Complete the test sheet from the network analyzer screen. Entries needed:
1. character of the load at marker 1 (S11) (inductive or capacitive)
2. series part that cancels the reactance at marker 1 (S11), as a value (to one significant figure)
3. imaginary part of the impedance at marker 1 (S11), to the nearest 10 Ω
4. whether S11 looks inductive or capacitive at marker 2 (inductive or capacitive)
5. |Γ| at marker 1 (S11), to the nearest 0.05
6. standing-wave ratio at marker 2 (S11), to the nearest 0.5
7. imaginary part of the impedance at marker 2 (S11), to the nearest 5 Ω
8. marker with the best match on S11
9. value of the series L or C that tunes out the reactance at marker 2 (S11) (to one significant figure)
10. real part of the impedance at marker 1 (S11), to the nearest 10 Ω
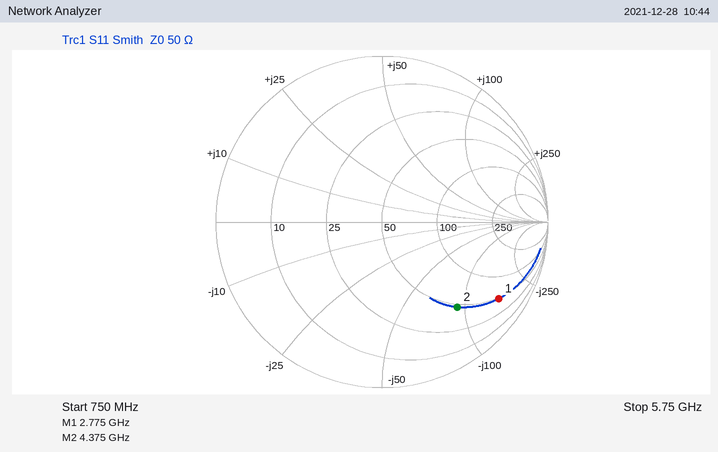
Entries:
capacitive
9 nH
-150 Ω
capacitive
0.85
5.5
-90 Ω
marker 2
3 nH
50 Ω
